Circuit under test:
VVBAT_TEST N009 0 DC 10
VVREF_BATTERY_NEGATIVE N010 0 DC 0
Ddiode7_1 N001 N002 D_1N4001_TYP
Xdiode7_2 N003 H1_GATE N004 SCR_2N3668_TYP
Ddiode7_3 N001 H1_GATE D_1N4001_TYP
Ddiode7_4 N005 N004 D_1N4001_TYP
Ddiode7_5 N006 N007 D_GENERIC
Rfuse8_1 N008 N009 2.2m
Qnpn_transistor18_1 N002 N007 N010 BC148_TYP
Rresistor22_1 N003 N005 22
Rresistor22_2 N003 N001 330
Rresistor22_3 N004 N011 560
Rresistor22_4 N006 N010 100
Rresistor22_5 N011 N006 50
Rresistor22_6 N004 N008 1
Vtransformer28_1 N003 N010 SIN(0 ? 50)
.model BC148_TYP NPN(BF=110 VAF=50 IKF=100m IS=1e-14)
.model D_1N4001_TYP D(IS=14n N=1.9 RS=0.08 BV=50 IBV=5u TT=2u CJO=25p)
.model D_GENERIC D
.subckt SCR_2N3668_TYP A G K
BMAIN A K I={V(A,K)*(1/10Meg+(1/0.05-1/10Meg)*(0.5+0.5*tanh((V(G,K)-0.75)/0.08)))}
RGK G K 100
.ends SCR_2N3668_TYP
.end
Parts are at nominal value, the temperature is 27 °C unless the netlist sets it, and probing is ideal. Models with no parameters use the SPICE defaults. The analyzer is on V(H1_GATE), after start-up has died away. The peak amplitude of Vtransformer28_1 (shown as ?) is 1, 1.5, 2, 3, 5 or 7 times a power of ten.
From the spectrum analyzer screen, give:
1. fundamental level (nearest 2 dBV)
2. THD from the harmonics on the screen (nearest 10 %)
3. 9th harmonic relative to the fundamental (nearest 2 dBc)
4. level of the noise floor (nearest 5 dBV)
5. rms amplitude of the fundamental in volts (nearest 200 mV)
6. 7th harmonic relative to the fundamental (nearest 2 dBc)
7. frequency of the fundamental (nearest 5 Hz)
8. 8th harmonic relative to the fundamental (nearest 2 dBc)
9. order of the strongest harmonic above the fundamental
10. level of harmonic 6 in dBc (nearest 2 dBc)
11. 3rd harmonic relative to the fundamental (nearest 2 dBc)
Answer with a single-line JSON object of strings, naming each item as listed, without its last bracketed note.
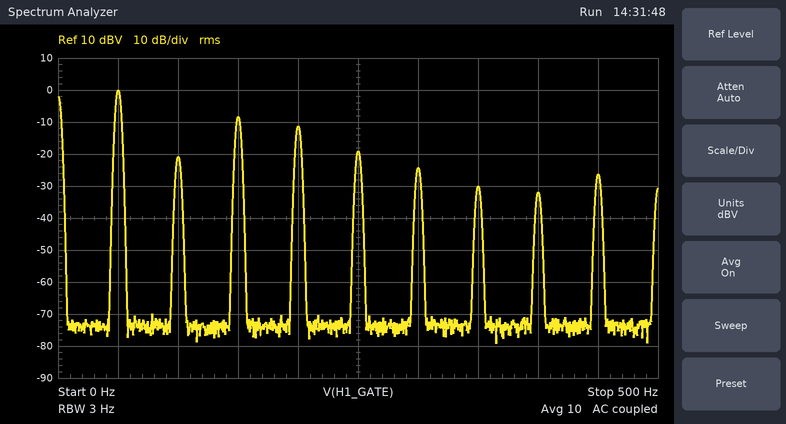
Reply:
{"fundamental level": "0 dBV", "THD from the harmonics on the screen": "50 %", "9th harmonic relative to the fundamental": "-26 dBc", "level of the noise floor": "-75 dBV", "rms amplitude of the fundamental in volts": "1.0 V", "7th harmonic relative to the fundamental": "-30 dBc", "frequency of the fundamental": "50 Hz", "8th harmonic relative to the fundamental": "-32 dBc", "order of the strongest harmonic above the fundamental": "3", "level of harmonic 6 in dBc": "-24 dBc", "3rd harmonic relative to the fundamental": "-8 dBc"}
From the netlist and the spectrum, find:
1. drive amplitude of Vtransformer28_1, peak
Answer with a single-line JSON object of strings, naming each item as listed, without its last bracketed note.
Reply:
{"drive amplitude of Vtransformer28_1, peak": "50 V"}
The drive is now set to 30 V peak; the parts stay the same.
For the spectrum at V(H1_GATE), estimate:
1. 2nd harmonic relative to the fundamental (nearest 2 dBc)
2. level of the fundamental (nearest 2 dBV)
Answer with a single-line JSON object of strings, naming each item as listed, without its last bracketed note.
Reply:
{"2nd harmonic relative to the fundamental": "-4 dBc", "level of the fundamental": "-12 dBV"}
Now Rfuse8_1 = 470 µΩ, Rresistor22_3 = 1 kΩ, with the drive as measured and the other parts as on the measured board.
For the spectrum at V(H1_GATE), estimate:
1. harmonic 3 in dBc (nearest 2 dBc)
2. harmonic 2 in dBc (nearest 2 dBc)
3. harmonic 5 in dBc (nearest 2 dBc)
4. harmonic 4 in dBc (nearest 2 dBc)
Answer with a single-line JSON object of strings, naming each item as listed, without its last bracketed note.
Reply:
{"harmonic 3 in dBc": "-50 dBc", "harmonic 2 in dBc": "-12 dBc", "harmonic 5 in dBc": "-38 dBc", "harmonic 4 in dBc": "-12 dBc"}
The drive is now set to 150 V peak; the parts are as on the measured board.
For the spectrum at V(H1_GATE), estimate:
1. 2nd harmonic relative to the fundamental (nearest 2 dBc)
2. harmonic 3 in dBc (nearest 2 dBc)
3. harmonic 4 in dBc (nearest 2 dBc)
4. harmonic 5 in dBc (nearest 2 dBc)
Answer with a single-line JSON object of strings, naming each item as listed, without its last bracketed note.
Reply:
{"2nd harmonic relative to the fundamental": "-14 dBc", "harmonic 3 in dBc": "-24 dBc", "harmonic 4 in dBc": "-22 dBc", "harmonic 5 in dBc": "-24 dBc"}
